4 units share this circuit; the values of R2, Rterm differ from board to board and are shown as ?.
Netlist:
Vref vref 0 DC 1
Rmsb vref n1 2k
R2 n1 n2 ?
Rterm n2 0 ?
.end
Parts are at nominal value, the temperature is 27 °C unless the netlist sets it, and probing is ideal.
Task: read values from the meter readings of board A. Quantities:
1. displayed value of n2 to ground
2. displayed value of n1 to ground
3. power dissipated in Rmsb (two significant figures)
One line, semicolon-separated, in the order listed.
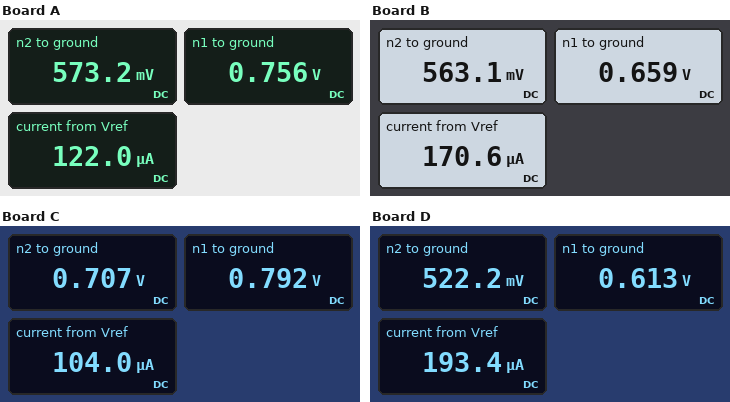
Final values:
573.2 mV; 0.756 V; 30 µW
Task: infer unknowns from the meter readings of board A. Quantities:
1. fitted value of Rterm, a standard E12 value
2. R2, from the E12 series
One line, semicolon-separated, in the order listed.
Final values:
4.7 kΩ; 1.5 kΩ
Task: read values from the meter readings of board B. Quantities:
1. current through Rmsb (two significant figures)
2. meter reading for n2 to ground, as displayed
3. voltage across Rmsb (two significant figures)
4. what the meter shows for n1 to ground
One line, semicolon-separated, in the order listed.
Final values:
170 µA; 563.1 mV; 340 mV; 0.659 V
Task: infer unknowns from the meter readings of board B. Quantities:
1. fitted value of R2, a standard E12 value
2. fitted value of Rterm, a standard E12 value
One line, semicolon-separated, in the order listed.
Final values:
560 Ω; 3.3 kΩ
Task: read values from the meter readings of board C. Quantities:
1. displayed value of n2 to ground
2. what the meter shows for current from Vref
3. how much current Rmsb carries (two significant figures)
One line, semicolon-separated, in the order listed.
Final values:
0.707 V; 104.0 µA; 100 µA
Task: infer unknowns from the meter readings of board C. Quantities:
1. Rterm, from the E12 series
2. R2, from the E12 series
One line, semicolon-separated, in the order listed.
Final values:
6.8 kΩ; 820 Ω
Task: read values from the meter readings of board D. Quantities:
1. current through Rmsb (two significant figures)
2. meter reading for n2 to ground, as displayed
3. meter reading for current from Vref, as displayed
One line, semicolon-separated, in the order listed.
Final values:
190 µA; 522.2 mV; 193.4 µA
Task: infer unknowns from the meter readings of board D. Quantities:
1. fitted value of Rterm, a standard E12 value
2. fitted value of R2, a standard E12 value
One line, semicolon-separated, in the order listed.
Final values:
2.7 kΩ; 470 Ω
